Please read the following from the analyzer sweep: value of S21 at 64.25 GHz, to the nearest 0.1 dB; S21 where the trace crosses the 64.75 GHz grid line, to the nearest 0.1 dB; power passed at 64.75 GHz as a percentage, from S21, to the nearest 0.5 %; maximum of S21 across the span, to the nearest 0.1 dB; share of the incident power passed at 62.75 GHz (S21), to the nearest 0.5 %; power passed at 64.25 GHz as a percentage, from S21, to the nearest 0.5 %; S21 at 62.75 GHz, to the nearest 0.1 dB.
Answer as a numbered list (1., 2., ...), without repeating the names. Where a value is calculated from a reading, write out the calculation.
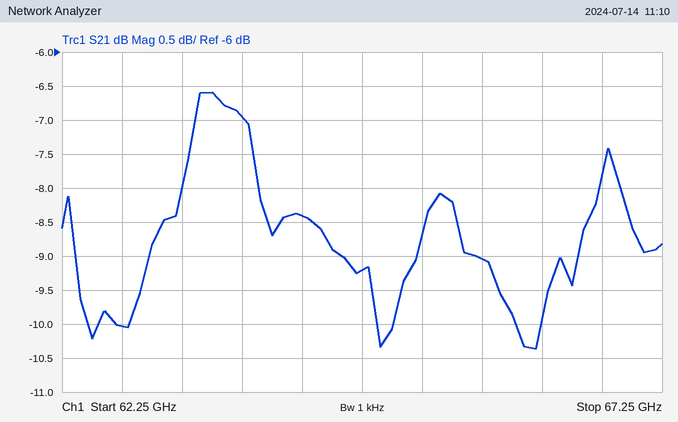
1. -8.4 dB
2. -9.2 dB
3. 10^(-9.2/10) ≈ 12.0 %
4. -6.6 dB
5. 10^(-10/10) ≈ 10.0 %
6. 10^(-8.4/10) ≈ 14.5 %
7. -10.0 dB
